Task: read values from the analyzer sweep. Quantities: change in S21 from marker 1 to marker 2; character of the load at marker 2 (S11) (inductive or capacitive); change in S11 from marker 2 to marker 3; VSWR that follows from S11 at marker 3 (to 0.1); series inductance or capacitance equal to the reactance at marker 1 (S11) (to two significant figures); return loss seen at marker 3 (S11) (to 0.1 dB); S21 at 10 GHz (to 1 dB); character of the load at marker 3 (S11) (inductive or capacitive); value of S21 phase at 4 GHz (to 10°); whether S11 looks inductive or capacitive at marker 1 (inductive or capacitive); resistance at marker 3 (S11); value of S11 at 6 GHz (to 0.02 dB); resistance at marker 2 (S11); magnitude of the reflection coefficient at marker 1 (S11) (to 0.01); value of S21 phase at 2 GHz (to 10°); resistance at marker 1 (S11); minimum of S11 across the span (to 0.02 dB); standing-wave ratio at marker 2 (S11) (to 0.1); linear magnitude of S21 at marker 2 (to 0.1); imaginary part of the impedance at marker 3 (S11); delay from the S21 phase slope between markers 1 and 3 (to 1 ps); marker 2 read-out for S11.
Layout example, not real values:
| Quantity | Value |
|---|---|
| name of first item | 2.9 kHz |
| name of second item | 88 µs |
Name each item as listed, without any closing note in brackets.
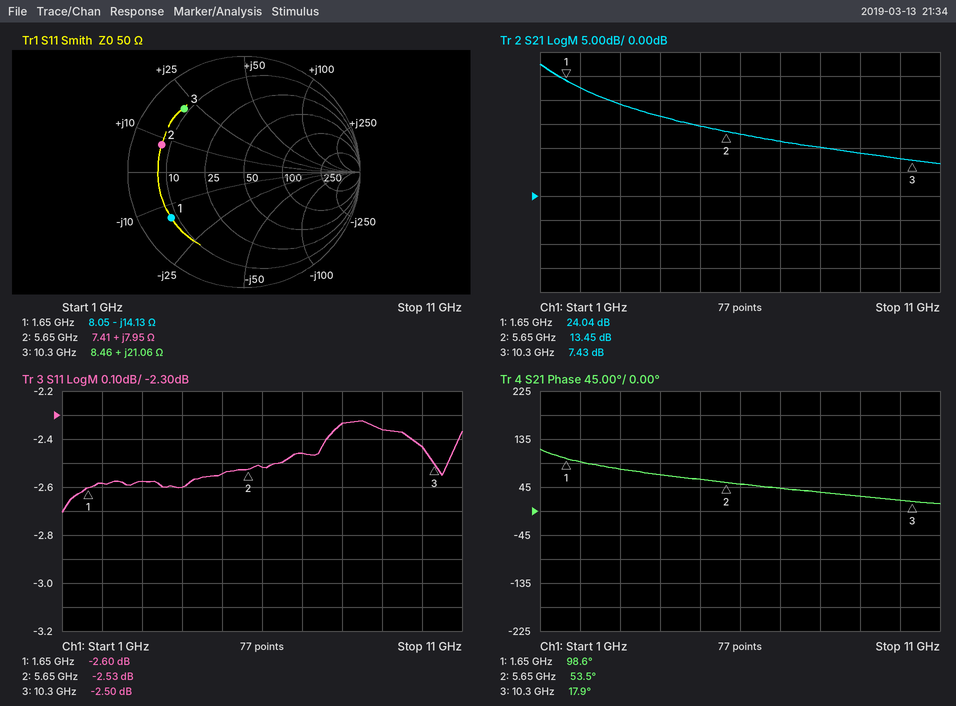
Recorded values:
| Quantity | Value |
|---|---|
| change in S21 from marker 1 to marker 2 | -10.59 dB |
| character of the load at marker 2 (S11) | inductive |
| change in S11 from marker 2 to marker 3 | 0.03 dB |
| VSWR that follows from S11 at marker 3 | 7.0 |
| series inductance or capacitance equal to the reactance at marker 1 (S11) | 6.8 pF |
| return loss seen at marker 3 (S11) | 2.5 dB |
| S21 at 10 GHz | 8 dB |
| character of the load at marker 3 (S11) | inductive |
| value of S21 phase at 4 GHz | 70° |
| whether S11 looks inductive or capacitive at marker 1 | capacitive |
| resistance at marker 3 | 8.46 Ω |
| value of S11 at 6 GHz | -2.52 dB |
| resistance at marker 2 | 7.41 Ω |
| magnitude of the reflection coefficient at marker 1 (S11) | 0.74 |
| value of S21 phase at 2 GHz | 90° |
| resistance at marker 1 | 8.05 Ω |
| minimum of S11 across the span | -2.70 dB |
| standing-wave ratio at marker 2 (S11) | 6.9 |
| linear magnitude of S21 at marker 2 | 4.7 |
| imaginary part of the impedance at marker 3 | +21.06 Ω |
| delay from the S21 phase slope between markers 1 and 3 | 26 ps |
| marker 2 read-out for S11 | -2.53 dB |
